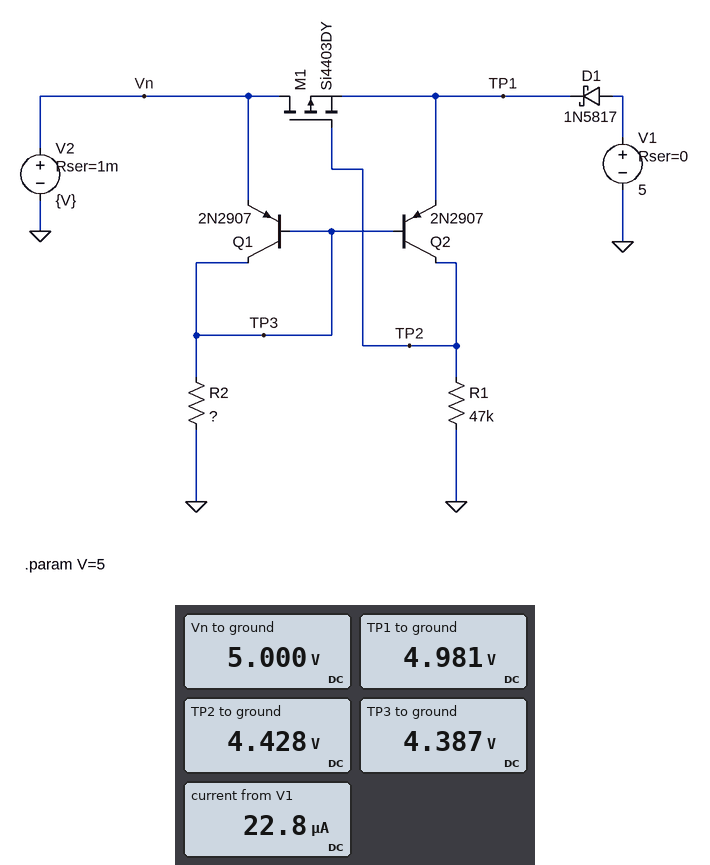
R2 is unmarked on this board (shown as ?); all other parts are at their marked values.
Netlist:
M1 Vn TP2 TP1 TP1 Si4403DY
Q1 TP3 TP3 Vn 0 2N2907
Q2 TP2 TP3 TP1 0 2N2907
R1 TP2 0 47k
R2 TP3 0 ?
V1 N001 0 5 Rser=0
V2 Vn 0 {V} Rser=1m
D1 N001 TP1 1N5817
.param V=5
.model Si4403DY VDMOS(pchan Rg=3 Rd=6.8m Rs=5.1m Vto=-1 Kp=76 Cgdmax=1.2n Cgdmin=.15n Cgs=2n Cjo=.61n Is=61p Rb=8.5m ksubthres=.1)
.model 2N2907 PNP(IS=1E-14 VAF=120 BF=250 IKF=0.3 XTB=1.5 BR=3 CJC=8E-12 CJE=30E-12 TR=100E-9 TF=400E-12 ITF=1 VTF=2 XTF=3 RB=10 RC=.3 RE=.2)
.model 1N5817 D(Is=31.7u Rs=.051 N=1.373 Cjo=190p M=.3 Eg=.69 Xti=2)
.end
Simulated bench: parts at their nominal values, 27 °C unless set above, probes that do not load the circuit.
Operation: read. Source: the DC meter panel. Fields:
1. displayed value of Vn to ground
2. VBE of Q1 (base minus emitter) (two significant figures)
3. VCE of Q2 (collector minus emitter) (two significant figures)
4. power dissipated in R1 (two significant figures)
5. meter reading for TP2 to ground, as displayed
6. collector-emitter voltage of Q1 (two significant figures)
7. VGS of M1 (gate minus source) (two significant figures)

5.000 V
-610 mV
-550 mV
420 µW
4.428 V
-610 mV
-550 mV
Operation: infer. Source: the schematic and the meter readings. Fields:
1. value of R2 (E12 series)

22 kΩ
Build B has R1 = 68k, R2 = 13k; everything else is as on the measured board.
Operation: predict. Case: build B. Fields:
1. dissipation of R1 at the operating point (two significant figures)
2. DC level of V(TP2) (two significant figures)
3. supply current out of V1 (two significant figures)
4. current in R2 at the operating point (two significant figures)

320 µW
4.7 V
69 µA
340 µA
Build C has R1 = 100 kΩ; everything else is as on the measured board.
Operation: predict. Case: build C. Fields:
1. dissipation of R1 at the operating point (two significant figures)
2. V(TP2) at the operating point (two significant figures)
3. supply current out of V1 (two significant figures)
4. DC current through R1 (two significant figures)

240 µW
4.9 V
50 µA
49 µA
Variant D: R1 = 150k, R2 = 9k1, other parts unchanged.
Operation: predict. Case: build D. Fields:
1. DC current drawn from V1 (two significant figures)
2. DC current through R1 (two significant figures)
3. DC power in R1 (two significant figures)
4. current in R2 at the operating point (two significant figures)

54 µA
33 µA
160 µW
480 µA
